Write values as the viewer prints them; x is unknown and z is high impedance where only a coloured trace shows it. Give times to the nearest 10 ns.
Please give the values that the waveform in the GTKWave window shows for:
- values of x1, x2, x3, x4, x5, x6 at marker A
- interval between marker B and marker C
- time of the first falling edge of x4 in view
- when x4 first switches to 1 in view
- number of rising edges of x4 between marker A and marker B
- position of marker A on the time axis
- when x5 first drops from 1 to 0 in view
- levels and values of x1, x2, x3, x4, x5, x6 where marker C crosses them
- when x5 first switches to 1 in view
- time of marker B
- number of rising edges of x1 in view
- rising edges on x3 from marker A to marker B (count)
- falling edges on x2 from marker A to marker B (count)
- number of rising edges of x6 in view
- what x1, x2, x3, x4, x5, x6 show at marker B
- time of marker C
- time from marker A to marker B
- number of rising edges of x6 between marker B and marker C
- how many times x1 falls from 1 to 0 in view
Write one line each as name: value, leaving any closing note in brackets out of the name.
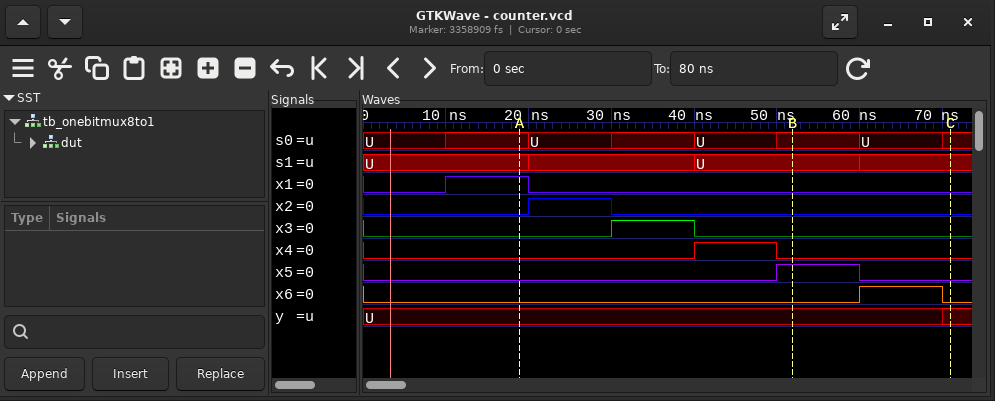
values of x1, x2, x3, x4, x5, x6 at marker A: x1=1, x2=0, x3=0, x4=0, x5=0, x6=0
interval between marker B and marker C: 20 ns
time of the first falling edge of x4 in view: 50 ns
when x4 first switches to 1 in view: 40 ns
number of rising edges of x4 between marker A and marker B: 1
position of marker A on the time axis: 20 ns
when x5 first drops from 1 to 0 in view: 60 ns
levels and values of x1, x2, x3, x4, x5, x6 where marker C crosses them: x1=0, x2=0, x3=0, x4=0, x5=0, x6=0
when x5 first switches to 1 in view: 50 ns
time of marker B: 50 ns
number of rising edges of x1 in view: 1
rising edges on x3 from marker A to marker B: 1
falling edges on x2 from marker A to marker B: 1
number of rising edges of x6 in view: 1
what x1, x2, x3, x4, x5, x6 show at marker B: x1=0, x2=0, x3=0, x4=0, x5=1, x6=0
time of marker C: 70 ns
time from marker A to marker B: 30 ns
number of rising edges of x6 between marker B and marker C: 1
how many times x1 falls from 1 to 0 in view: 1
